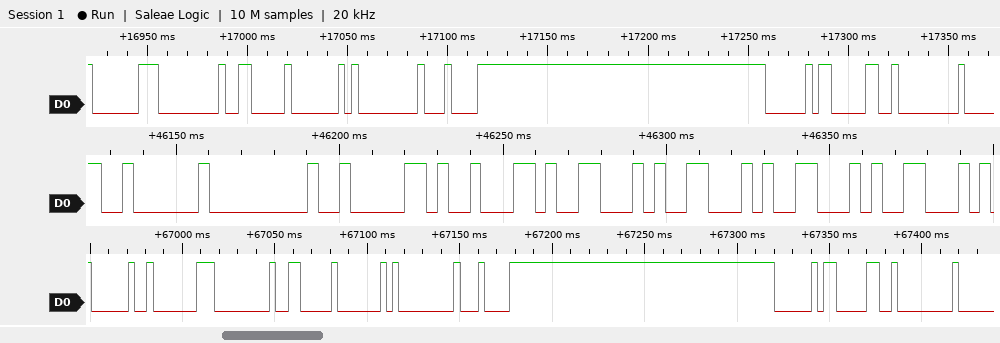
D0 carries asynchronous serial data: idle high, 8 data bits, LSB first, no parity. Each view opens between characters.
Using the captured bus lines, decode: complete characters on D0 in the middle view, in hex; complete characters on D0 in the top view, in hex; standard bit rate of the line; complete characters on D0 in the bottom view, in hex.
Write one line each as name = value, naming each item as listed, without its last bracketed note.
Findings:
complete characters on D0 in the middle view, in hex = 02, 00, 82, 89, 19, 19, 19, 19
complete characters on D0 in the top view, in hex = C0, 00, 06, 40, 00, 84, A0, 30, 00
standard bit rate of the line = 300 baud
complete characters on D0 in the bottom view, in hex = 20, C0, 00, 06, 40, 00, 84, A0, 30, 00
